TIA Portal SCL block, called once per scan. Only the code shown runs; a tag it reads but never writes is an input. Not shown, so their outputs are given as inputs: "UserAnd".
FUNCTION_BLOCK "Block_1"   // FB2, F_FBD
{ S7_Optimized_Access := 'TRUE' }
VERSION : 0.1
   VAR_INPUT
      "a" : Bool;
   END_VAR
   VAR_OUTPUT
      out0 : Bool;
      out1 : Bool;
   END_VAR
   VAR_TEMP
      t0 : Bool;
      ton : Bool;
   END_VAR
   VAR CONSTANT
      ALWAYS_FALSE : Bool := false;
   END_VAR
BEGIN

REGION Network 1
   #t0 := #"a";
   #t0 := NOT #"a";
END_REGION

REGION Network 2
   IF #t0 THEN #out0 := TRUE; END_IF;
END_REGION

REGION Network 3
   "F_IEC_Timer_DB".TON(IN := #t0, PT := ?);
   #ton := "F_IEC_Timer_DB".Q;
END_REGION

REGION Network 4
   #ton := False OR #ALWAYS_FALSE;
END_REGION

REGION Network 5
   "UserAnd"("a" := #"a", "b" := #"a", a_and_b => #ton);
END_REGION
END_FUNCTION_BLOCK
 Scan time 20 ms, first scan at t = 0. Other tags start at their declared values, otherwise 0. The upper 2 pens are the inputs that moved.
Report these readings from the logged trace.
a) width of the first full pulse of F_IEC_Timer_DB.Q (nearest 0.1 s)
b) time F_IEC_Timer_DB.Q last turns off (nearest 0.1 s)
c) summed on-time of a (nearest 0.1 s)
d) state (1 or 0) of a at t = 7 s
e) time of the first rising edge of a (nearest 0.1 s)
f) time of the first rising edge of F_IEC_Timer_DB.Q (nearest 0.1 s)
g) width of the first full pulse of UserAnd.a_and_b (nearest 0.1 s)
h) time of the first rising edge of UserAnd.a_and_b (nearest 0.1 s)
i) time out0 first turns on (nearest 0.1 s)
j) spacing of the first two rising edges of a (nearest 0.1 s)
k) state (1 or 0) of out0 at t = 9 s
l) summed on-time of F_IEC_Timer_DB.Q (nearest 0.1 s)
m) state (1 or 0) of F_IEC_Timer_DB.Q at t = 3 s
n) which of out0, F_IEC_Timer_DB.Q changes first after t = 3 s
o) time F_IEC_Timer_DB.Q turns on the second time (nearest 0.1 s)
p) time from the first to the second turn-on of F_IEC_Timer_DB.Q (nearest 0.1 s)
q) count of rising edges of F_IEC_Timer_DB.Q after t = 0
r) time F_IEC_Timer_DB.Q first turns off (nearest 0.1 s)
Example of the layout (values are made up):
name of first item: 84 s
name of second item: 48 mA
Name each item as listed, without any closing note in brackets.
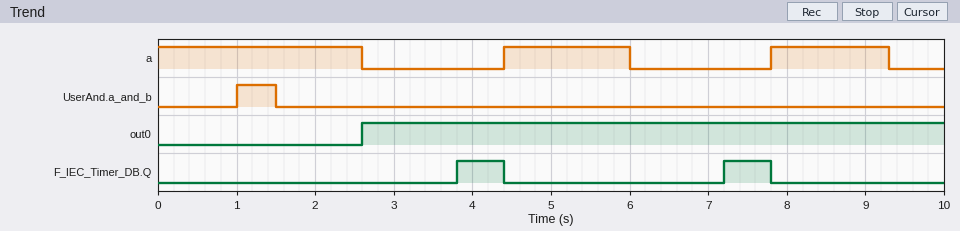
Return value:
width of the first full pulse of F_IEC_Timer_DB.Q: 0.6 s
time F_IEC_Timer_DB.Q last turns off: 7.8 s
summed on-time of a: 5.7 s
state (1 or 0) of a at t = 7 s: 0
time of the first rising edge of a: 4.4 s
time of the first rising edge of F_IEC_Timer_DB.Q: 3.8 s
width of the first full pulse of UserAnd.a_and_b: 0.5 s
time of the first rising edge of UserAnd.a_and_b: 1.0 s
time out0 first turns on: 2.6 s
spacing of the first two rising edges of a: 3.4 s
state (1 or 0) of out0 at t = 9 s: 1
summed on-time of F_IEC_Timer_DB.Q: 1.2 s
state (1 or 0) of F_IEC_Timer_DB.Q at t = 3 s: 0
which of out0, F_IEC_Timer_DB.Q changes first after t = 3 s: F_IEC_Timer_DB.Q
time F_IEC_Timer_DB.Q turns on the second time: 7.2 s
time from the first to the second turn-on of F_IEC_Timer_DB.Q: 3.4 s
count of rising edges of F_IEC_Timer_DB.Q after t = 0: 2
time F_IEC_Timer_DB.Q first turns off: 4.4 s
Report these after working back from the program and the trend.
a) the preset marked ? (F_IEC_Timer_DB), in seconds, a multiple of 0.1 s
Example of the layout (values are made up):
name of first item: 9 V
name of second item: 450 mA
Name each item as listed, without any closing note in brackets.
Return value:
the preset marked ? (F_IEC_Timer_DB), in seconds, a multiple of 0.1 s: 1.2 s
